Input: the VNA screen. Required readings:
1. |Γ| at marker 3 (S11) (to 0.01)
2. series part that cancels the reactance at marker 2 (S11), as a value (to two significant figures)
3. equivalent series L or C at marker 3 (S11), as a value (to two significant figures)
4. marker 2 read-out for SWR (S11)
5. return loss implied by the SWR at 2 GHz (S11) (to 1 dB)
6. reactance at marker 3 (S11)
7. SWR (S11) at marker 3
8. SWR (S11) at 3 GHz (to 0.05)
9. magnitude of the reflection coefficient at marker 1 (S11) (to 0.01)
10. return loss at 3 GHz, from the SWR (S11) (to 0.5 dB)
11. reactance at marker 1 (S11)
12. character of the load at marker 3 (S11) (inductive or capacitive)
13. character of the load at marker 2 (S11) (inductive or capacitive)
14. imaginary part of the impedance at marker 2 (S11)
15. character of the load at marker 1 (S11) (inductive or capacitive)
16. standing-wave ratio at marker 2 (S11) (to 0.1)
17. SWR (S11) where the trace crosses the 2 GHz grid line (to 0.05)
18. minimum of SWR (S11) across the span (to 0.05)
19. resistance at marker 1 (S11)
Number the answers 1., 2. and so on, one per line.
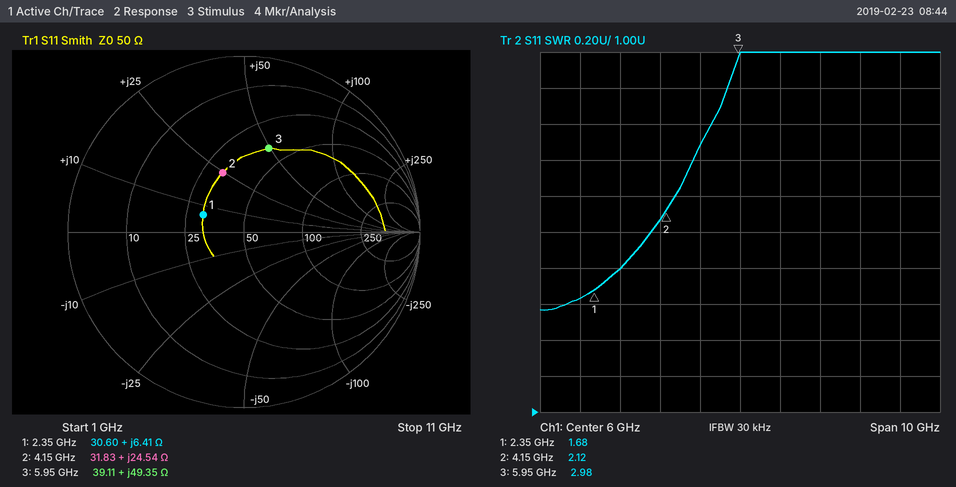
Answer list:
1. 0.50
2. 1.6 pF
3. 1.3 nH
4. 2.12
5. 12 dB
6. +49.35 Ω
7. 2.98
8. 1.80
9. 0.25
10. 11.0 dB
11. +6.41 Ω
12. inductive
13. inductive
14. +24.54 Ω
15. inductive
16. 2.1
17. 1.65
18. 1.55
19. 30.60 Ω
